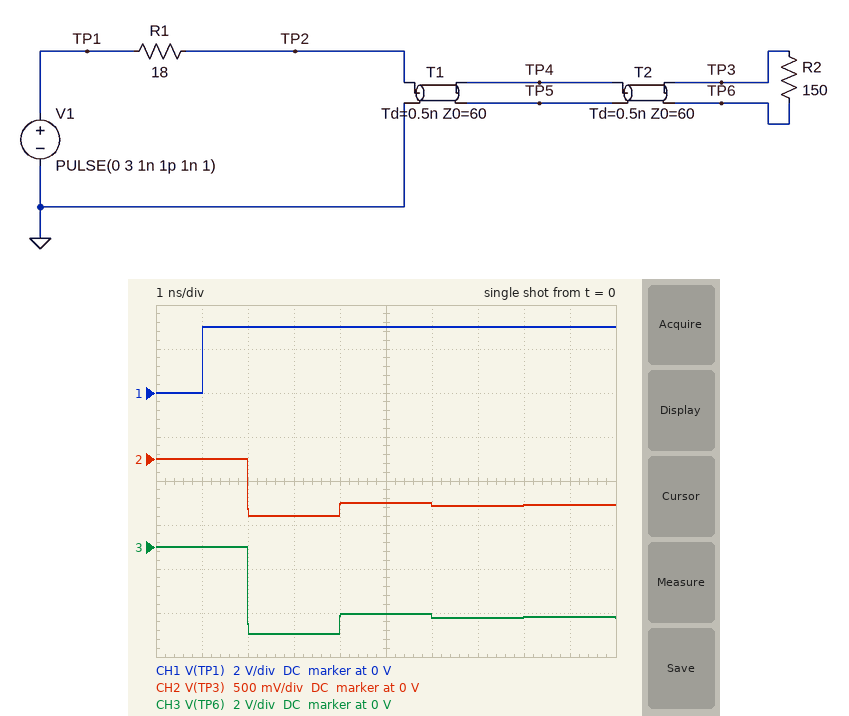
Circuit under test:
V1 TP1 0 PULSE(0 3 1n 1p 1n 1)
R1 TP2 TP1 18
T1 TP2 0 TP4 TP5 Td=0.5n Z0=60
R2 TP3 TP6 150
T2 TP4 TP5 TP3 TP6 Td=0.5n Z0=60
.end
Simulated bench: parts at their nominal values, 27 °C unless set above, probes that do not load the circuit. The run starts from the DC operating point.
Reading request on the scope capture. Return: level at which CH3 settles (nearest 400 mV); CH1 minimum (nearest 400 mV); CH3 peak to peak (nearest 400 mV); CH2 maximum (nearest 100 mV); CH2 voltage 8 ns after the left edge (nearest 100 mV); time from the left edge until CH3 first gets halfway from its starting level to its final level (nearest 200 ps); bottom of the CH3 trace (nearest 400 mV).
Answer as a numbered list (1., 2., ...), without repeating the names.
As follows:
1. -3.2 V
2. 0 V
3. 4.0 V
4. 0 V
5. -500 mV
6. 2.0 ns
7. -4.0 V
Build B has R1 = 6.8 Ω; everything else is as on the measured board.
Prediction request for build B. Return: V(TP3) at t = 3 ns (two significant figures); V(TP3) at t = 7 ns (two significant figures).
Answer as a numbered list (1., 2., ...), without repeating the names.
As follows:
1. -760 mV
2. -590 mV
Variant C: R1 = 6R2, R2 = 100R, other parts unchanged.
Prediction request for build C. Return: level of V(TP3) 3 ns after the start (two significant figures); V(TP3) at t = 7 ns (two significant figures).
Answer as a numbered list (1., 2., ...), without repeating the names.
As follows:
1. -1.0 V
2. -840 mV
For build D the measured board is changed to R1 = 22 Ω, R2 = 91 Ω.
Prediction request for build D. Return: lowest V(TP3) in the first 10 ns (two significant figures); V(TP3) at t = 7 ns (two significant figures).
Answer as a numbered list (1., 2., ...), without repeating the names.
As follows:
1. -860 mV
2. -780 mV
